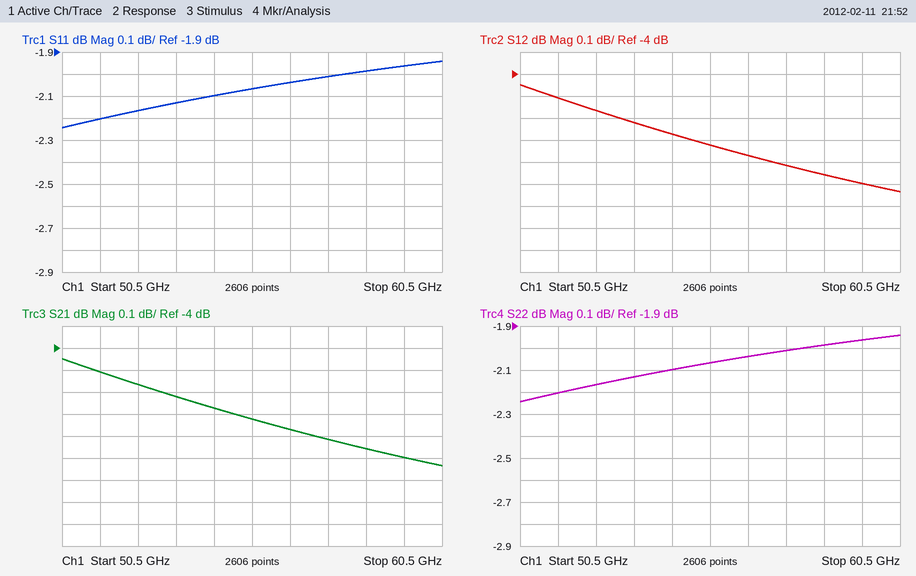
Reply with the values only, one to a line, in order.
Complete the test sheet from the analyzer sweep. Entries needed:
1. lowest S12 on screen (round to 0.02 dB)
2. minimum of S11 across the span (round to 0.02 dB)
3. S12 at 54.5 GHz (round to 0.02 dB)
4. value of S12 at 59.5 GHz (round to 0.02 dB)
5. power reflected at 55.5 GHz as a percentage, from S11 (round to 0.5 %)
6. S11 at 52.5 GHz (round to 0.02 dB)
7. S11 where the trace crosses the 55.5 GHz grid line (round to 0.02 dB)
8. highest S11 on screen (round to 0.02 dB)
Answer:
-4.54 dB
-2.24 dB
-4.28 dB
-4.50 dB
62.0 %
-2.16 dB
-2.06 dB
-1.94 dB
